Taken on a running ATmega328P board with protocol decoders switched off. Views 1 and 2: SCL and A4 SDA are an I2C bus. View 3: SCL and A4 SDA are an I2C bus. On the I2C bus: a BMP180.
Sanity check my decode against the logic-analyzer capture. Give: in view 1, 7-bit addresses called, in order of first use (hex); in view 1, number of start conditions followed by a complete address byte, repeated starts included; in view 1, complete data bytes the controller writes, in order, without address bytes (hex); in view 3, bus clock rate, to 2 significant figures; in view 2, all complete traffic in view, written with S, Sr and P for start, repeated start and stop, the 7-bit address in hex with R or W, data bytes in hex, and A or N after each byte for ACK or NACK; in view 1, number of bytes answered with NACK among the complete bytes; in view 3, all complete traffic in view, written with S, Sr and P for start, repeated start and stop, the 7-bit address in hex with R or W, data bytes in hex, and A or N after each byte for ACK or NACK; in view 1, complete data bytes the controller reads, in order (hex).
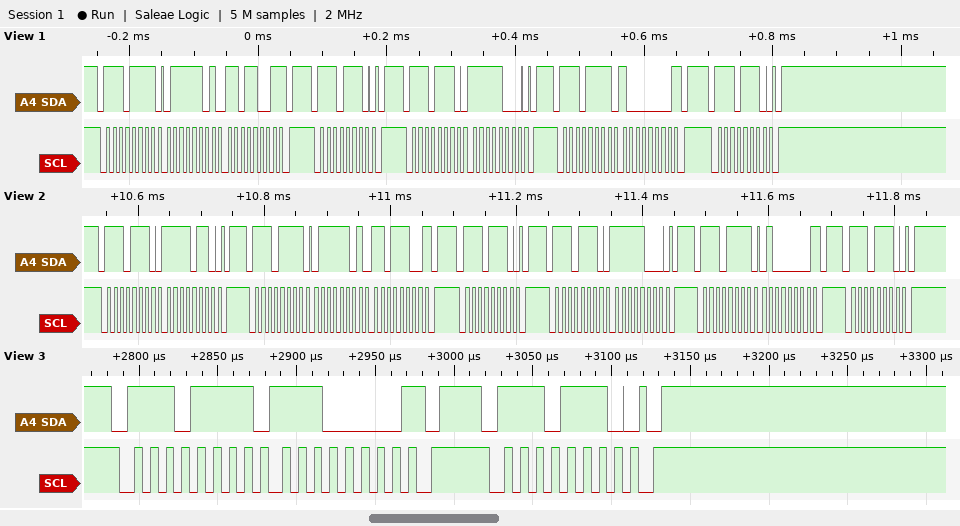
0x77
5
F8
100 kHz
S 77W A F6 A P S 77R A 7D A DC N P S 77W A P S 77W A F8 A P S 77R A 40 N P S 77W A P
2
S 77R A E0 N P S 77W A P
7D D9 80
